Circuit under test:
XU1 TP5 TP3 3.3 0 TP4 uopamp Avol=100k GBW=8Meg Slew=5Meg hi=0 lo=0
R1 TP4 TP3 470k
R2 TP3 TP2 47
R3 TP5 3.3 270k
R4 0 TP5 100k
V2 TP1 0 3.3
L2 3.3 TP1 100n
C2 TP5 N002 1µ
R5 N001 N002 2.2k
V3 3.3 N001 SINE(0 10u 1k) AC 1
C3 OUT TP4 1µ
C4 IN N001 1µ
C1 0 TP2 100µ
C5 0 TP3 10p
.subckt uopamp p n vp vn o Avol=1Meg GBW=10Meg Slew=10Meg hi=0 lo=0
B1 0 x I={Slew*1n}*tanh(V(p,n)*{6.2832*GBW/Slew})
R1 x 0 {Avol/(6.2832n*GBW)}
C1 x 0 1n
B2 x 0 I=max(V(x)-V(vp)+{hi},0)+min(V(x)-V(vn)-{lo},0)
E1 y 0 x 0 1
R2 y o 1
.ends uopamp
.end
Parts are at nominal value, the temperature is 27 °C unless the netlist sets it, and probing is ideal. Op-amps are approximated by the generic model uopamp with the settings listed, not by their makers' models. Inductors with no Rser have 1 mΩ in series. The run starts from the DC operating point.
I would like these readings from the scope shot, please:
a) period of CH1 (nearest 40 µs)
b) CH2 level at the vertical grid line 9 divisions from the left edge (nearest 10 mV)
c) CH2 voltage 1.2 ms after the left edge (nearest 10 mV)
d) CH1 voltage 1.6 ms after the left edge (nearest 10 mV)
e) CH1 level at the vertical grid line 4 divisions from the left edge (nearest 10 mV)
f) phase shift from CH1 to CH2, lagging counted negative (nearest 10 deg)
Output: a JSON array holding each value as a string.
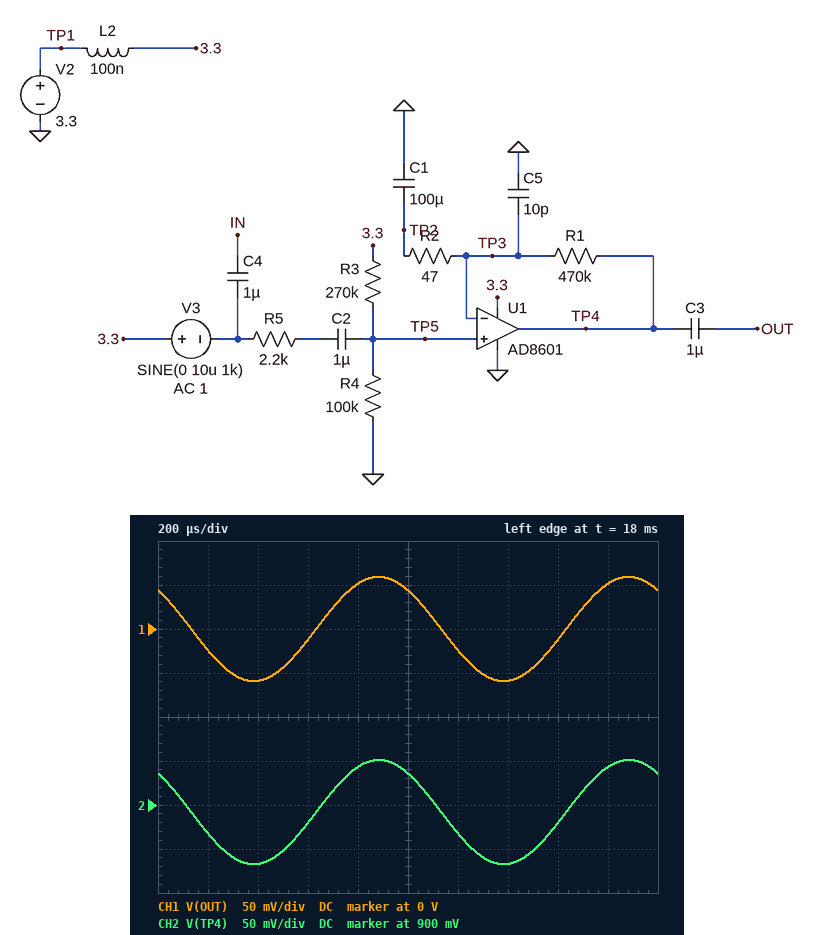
["1.00 ms", "940 mV", "870 mV", "-10 mV", "50 mV", "0 deg"]
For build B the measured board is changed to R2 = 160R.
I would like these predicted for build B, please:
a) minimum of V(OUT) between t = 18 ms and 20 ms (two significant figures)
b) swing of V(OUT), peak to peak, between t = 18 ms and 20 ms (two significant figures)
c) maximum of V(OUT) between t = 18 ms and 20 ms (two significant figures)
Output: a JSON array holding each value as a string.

["-26 mV", "52 mV", "26 mV"]
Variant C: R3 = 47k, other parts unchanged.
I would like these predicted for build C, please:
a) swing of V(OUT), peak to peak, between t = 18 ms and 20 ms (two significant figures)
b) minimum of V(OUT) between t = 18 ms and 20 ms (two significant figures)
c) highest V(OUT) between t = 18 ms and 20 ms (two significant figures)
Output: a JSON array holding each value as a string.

["110 mV", "-57 mV", "57 mV"]
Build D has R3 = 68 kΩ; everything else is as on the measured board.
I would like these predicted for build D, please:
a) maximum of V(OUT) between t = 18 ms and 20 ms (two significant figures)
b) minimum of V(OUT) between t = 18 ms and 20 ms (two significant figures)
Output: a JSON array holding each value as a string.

["58 mV", "-58 mV"]
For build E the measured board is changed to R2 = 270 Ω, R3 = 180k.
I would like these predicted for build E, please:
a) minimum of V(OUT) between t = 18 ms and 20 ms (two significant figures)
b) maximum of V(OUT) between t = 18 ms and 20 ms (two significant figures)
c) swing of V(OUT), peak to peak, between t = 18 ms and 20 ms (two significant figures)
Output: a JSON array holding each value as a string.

["-16 mV", "16 mV", "32 mV"]
